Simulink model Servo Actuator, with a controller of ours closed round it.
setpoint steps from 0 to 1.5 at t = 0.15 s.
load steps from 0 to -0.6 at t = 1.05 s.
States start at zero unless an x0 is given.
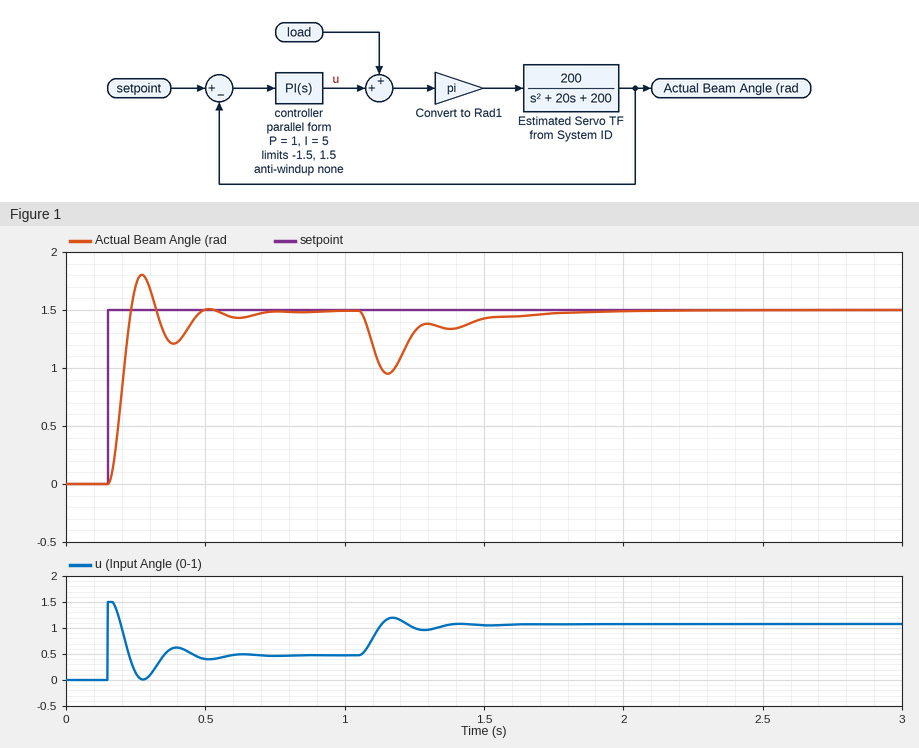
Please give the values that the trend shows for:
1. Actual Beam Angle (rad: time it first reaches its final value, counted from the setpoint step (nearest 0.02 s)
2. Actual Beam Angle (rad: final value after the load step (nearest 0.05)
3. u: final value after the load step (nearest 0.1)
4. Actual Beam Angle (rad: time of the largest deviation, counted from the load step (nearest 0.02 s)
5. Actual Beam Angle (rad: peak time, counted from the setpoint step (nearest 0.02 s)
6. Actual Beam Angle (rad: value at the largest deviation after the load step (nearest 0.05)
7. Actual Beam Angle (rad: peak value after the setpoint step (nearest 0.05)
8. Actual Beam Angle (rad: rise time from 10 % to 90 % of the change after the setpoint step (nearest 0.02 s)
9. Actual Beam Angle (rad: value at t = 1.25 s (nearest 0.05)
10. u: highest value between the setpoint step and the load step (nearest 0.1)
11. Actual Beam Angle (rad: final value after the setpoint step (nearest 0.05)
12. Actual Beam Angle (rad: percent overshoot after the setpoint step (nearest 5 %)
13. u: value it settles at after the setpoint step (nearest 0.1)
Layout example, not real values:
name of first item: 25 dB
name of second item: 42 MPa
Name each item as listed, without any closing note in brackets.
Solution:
Actual Beam Angle (rad: time it first reaches its final value, counted from the setpoint step: 0.08 s
Actual Beam Angle (rad: final value after the load step: 1.50
u: final value after the load step: 1.1
Actual Beam Angle (rad: time of the largest deviation, counted from the load step: 0.10 s
Actual Beam Angle (rad: peak time, counted from the setpoint step: 0.12 s
Actual Beam Angle (rad: value at the largest deviation after the load step: 0.95
Actual Beam Angle (rad: peak value after the setpoint step: 1.80
Actual Beam Angle (rad: rise time from 10 % to 90 % of the change after the setpoint step: 0.06 s
Actual Beam Angle (rad: value at t = 1.25 s: 1.30
u: highest value between the setpoint step and the load step: 1.5
Actual Beam Angle (rad: final value after the setpoint step: 1.50
Actual Beam Angle (rad: percent overshoot after the setpoint step: 20 %
u: value it settles at after the setpoint step: 0.5
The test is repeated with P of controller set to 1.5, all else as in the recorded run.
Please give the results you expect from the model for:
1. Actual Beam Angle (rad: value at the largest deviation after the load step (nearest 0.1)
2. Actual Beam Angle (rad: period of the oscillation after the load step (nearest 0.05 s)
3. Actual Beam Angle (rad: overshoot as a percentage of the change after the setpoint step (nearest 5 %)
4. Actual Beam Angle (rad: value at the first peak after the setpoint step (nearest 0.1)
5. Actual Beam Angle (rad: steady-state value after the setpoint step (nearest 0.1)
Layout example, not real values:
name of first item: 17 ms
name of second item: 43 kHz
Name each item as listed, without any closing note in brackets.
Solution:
Actual Beam Angle (rad: value at the largest deviation after the load step: 1.1
Actual Beam Angle (rad: period of the oscillation after the load step: 0.20 s
Actual Beam Angle (rad: overshoot as a percentage of the change after the setpoint step: 25 %
Actual Beam Angle (rad: value at the first peak after the setpoint step: 1.9
Actual Beam Angle (rad: steady-state value after the setpoint step: 1.5
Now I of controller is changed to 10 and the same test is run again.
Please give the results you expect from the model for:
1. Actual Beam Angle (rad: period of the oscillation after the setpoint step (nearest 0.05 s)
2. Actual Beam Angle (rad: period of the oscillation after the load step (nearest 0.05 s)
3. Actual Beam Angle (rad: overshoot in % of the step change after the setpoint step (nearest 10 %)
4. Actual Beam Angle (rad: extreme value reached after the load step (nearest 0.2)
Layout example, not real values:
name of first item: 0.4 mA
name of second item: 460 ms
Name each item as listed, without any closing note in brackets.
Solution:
Actual Beam Angle (rad: period of the oscillation after the setpoint step: 0.25 s
Actual Beam Angle (rad: period of the oscillation after the load step: 0.25 s
Actual Beam Angle (rad: overshoot in % of the step change after the setpoint step: 40 %
Actual Beam Angle (rad: extreme value reached after the load step: 1.0
